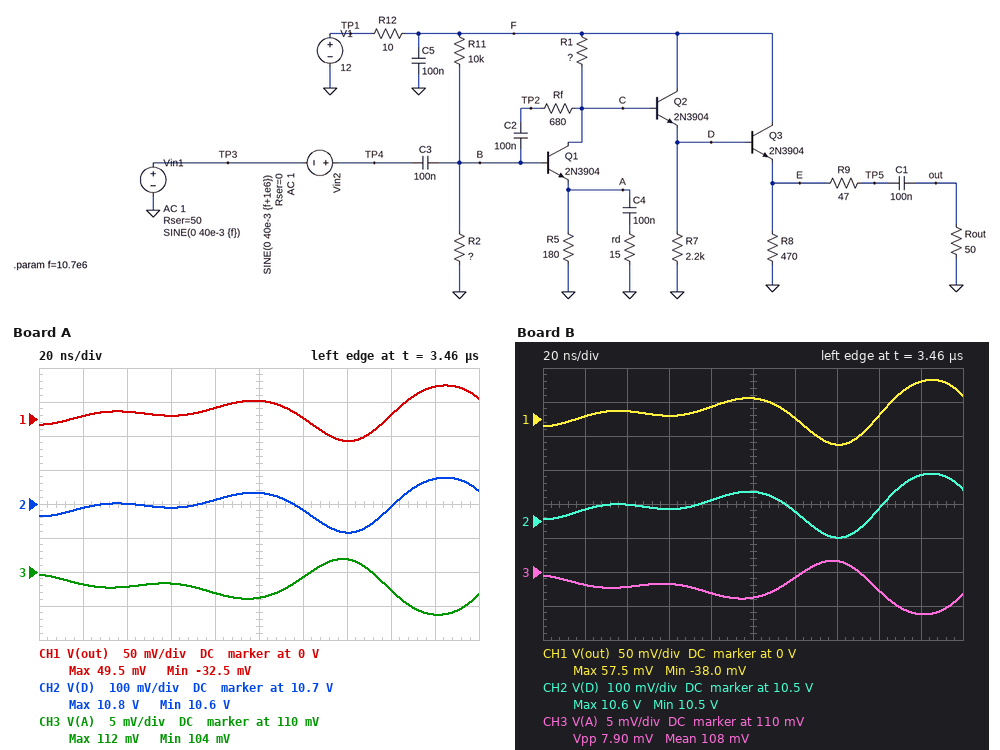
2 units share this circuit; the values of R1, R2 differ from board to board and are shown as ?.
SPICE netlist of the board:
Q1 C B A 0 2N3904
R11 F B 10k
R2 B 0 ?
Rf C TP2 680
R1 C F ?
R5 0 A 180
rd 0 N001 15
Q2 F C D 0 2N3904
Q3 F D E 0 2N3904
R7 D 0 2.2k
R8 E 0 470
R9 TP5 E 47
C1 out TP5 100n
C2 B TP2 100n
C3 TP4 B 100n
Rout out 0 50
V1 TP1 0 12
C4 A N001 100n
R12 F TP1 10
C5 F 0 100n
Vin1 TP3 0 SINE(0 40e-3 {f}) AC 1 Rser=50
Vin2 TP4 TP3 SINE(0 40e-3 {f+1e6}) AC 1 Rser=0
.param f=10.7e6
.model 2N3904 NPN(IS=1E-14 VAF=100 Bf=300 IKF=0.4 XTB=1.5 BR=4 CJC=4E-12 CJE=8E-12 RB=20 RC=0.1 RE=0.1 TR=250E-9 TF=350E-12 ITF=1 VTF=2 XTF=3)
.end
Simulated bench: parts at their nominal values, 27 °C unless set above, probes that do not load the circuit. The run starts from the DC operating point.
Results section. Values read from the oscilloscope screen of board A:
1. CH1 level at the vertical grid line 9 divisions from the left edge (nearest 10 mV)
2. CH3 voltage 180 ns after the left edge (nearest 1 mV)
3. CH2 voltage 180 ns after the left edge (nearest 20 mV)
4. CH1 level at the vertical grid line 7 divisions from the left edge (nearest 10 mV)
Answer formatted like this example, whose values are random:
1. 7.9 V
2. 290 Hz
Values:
1. 50 mV
2. 104 mV
3. 10.78 V
4. -30 mV
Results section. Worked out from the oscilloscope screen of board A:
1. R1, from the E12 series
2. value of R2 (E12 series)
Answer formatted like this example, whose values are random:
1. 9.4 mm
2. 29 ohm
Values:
1. 560 Ω
2. 680 Ω
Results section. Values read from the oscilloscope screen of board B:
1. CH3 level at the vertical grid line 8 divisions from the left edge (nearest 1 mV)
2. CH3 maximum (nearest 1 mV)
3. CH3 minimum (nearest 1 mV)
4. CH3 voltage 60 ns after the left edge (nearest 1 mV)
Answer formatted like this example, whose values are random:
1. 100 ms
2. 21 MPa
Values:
1. 107 mV
2. 112 mV
3. 104 mV
4. 108 mV
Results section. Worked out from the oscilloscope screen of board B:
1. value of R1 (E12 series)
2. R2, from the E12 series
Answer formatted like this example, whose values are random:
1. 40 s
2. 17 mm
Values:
1. 820 Ω
2. 680 Ω
